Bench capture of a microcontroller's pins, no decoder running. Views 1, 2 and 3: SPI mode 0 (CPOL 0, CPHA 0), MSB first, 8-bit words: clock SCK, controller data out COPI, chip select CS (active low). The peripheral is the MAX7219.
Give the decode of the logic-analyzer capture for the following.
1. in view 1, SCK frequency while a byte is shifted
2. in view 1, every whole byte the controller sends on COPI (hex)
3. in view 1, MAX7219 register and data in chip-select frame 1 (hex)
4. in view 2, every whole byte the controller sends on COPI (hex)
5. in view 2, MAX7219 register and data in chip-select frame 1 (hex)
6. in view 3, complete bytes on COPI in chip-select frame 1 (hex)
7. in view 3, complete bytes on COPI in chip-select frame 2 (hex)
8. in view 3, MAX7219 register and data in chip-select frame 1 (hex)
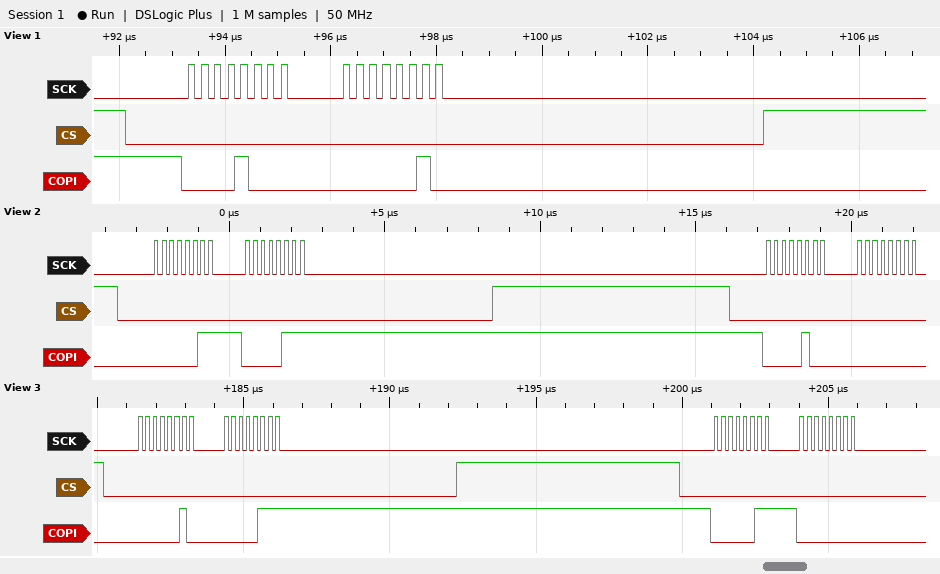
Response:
4 MHz
0x08 0x02
register 0x8, data 0x02
0x03 0x07 0x04 0x00
register 0x3, data 0x07
02 07
03 00
register 0x2, data 0x07
